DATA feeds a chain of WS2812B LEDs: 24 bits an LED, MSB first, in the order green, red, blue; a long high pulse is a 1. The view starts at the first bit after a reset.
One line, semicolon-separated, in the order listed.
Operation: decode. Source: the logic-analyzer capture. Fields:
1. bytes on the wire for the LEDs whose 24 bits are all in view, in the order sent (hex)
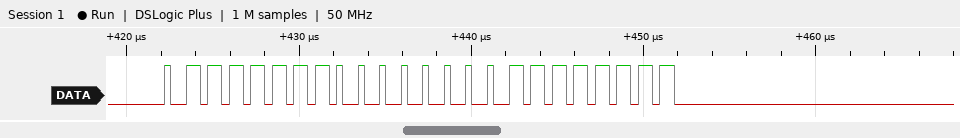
7F 00 FF
